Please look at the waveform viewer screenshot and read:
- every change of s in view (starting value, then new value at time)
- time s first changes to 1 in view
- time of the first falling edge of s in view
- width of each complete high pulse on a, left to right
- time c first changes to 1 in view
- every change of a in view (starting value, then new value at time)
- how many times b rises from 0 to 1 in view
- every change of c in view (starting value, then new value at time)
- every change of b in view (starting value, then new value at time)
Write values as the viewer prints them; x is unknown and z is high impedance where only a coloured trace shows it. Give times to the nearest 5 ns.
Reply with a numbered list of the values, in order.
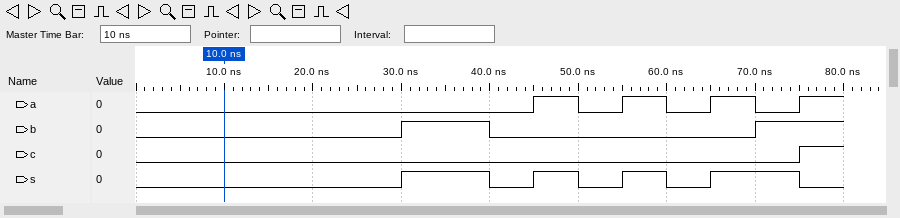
1. 0, 1 at 30 ns, 0 at 40 ns, 1 at 45 ns, 0 at 50 ns, 1 at 55 ns, 0 at 60 ns, 1 at 65 ns, 0 at 75 ns
2. 30 ns
3. 40 ns
4. 5 ns, 5 ns, 5 ns
5. 75 ns
6. 0, 1 at 45 ns, 0 at 50 ns, 1 at 55 ns, 0 at 60 ns, 1 at 65 ns, 0 at 70 ns, 1 at 75 ns
7. 2
8. 0, 1 at 75 ns
9. 0, 1 at 30 ns, 0 at 40 ns, 1 at 70 ns
